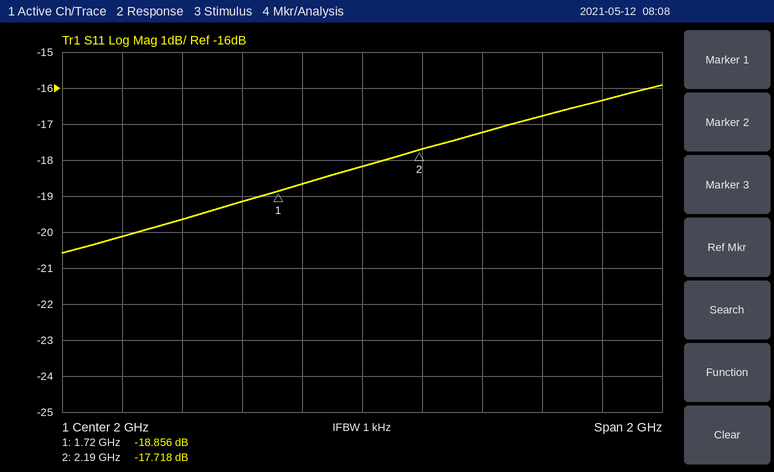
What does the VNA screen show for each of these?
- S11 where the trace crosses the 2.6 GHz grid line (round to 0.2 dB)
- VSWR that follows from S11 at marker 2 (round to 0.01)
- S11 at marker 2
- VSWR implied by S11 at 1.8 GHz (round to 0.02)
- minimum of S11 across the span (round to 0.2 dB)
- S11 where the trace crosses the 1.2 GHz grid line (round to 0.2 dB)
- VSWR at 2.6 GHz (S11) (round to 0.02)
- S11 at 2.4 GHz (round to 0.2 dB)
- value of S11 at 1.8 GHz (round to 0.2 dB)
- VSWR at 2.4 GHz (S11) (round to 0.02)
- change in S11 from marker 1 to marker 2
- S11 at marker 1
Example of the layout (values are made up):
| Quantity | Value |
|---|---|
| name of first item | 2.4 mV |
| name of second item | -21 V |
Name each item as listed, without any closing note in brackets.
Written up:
| Quantity | Value |
|---|---|
| S11 where the trace crosses the 2.6 GHz grid line | -16.8 dB |
| VSWR that follows from S11 at marker 2 | 1.30 |
| S11 at marker 2 | -17.718 dB |
| VSWR implied by S11 at 1.8 GHz | 1.26 |
| minimum of S11 across the span | -20.6 dB |
| S11 where the trace crosses the 1.2 GHz grid line | -20.2 dB |
| VSWR at 2.6 GHz (S11) | 1.34 |
| S11 at 2.4 GHz | -17.2 dB |
| value of S11 at 1.8 GHz | -18.6 dB |
| VSWR at 2.4 GHz (S11) | 1.32 |
| change in S11 from marker 1 to marker 2 | 1.138 dB |
| S11 at marker 1 | -18.856 dB |
